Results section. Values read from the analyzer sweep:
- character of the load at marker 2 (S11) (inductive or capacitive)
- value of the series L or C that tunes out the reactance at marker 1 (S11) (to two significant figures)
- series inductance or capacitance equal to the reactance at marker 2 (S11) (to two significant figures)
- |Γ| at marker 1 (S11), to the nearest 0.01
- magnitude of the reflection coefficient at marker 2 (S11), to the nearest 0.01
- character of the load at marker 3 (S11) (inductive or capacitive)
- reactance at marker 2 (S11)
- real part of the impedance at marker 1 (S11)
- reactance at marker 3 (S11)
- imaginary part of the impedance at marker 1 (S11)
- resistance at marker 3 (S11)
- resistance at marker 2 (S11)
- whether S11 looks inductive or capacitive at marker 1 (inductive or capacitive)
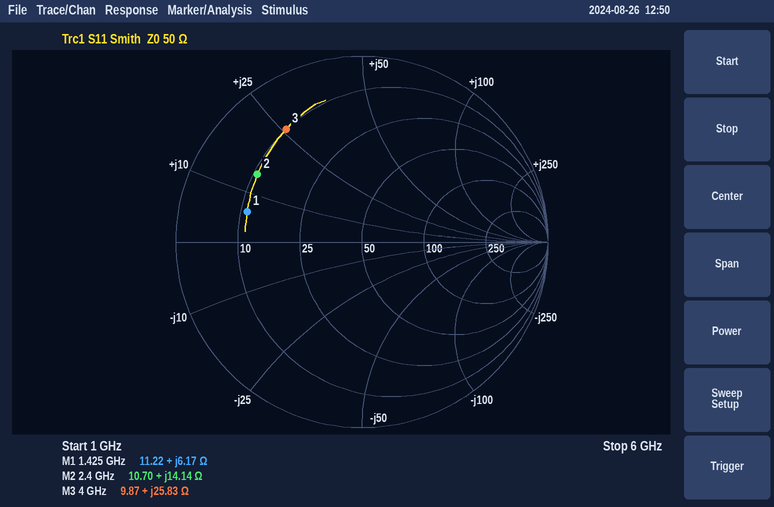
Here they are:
inductive
18 pF
940 pH
0.64
0.67
inductive
+14.14 Ω
11.22 Ω
+25.83 Ω
+6.17 Ω
9.87 Ω
10.70 Ω
inductive
